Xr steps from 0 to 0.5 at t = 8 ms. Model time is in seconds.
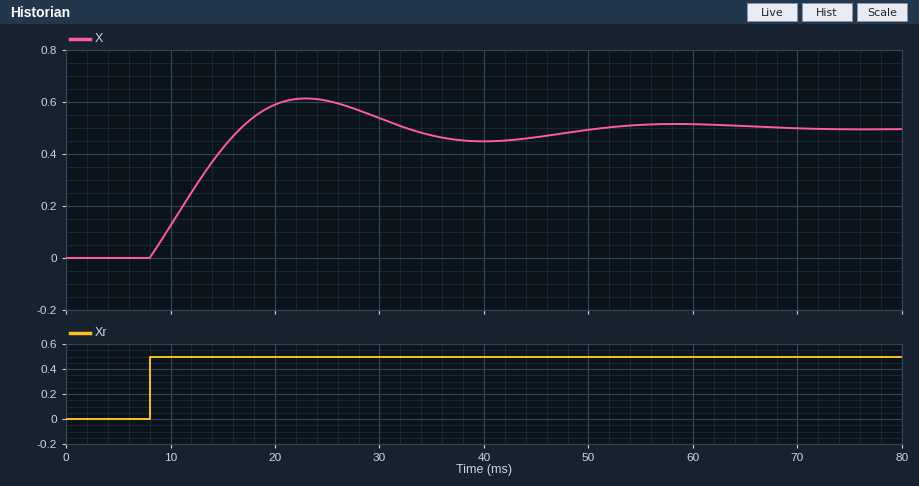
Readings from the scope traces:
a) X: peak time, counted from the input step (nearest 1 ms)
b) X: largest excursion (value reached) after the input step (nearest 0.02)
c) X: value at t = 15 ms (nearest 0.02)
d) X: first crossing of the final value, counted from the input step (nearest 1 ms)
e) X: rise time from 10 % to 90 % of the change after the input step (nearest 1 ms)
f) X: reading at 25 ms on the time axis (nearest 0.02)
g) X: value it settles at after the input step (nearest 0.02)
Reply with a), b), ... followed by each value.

a) 15 ms
b) 0.62
c) 0.42
d) 9 ms
e) 7 ms
f) 0.60
g) 0.50
